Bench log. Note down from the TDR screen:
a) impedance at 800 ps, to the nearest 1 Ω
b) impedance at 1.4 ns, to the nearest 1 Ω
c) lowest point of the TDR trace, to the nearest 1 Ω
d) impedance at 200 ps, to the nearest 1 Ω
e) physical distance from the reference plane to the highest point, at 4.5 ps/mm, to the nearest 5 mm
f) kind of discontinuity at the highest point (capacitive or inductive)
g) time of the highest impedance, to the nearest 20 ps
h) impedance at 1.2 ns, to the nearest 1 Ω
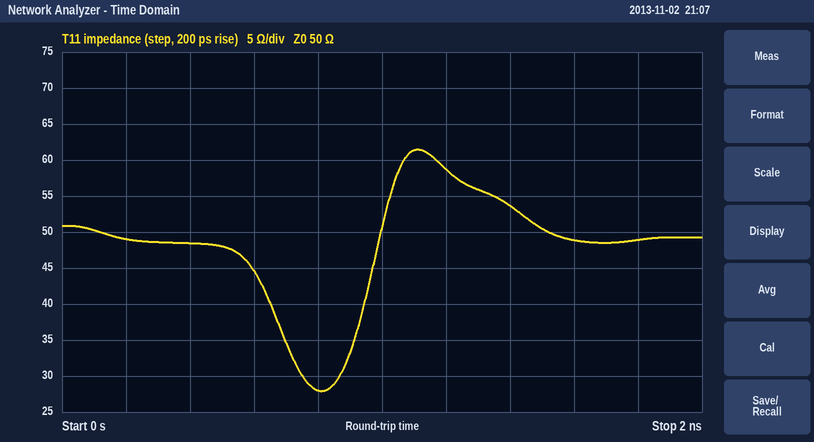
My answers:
28 Ω
54 Ω
28 Ω
49 Ω
125 mm
inductive
1.12 ns
59 Ω
